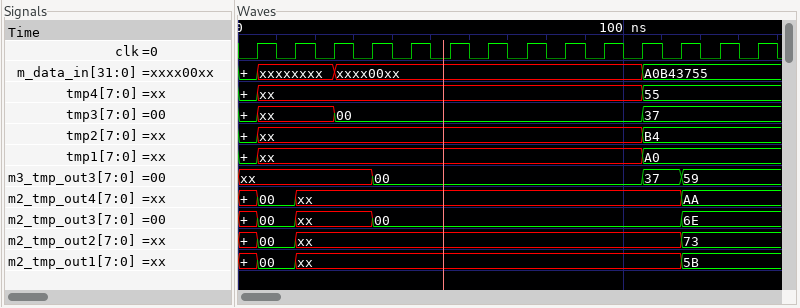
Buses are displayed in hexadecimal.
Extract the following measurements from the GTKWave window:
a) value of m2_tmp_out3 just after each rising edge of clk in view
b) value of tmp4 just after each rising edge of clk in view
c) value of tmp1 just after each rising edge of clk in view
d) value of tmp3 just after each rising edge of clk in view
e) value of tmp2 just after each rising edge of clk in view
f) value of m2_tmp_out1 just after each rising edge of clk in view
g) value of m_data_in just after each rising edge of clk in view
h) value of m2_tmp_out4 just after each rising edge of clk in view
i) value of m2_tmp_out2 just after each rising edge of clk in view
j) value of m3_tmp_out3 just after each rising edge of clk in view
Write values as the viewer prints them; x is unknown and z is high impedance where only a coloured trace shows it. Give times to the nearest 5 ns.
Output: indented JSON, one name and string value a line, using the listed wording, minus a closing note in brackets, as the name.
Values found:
{
  "value of m2_tmp_out3 just after each rising edge of clk in view": "00, xx, xx, 00, 00, 00, 00, 00, 00, 00, 00, 6E, 6E, 6E",
  "value of tmp4 just after each rising edge of clk in view": "xx, xx, xx, xx, xx, xx, xx, xx, xx, xx, 55, 55, 55, 55",
  "value of tmp1 just after each rising edge of clk in view": "xx, xx, xx, xx, xx, xx, xx, xx, xx, xx, A0, A0, A0, A0",
  "value of tmp3 just after each rising edge of clk in view": "xx, xx, 00, 00, 00, 00, 00, 00, 00, 00, 37, 37, 37, 37",
  "value of tmp2 just after each rising edge of clk in view": "xx, xx, xx, xx, xx, xx, xx, xx, xx, xx, B4, B4, B4, B4",
  "value of m2_tmp_out1 just after each rising edge of clk in view": "00, xx, xx, xx, xx, xx, xx, xx, xx, xx, xx, 5B, 5B, 5B",
  "value of m_data_in just after each rising edge of clk in view": "xxxxxxxx, xxxxxxxx, xxxx00xx, xxxx00xx, xxxx00xx, xxxx00xx, xxxx00xx, xxxx00xx, xxxx00xx, xxxx00xx, A0B43755, A0B43755, A0B43755, A0B43755",
  "value of m2_tmp_out4 just after each rising edge of clk in view": "00, xx, xx, xx, xx, xx, xx, xx, xx, xx, xx, AA, AA, AA",
  "value of m2_tmp_out2 just after each rising edge of clk in view": "00, xx, xx, xx, xx, xx, xx, xx, xx, xx, xx, 73, 73, 73",
  "value of m3_tmp_out3 just after each rising edge of clk in view": "xx, xx, xx, 00, 00, 00, 00, 00, 00, 00, 37, 59, 59, 59"
}
